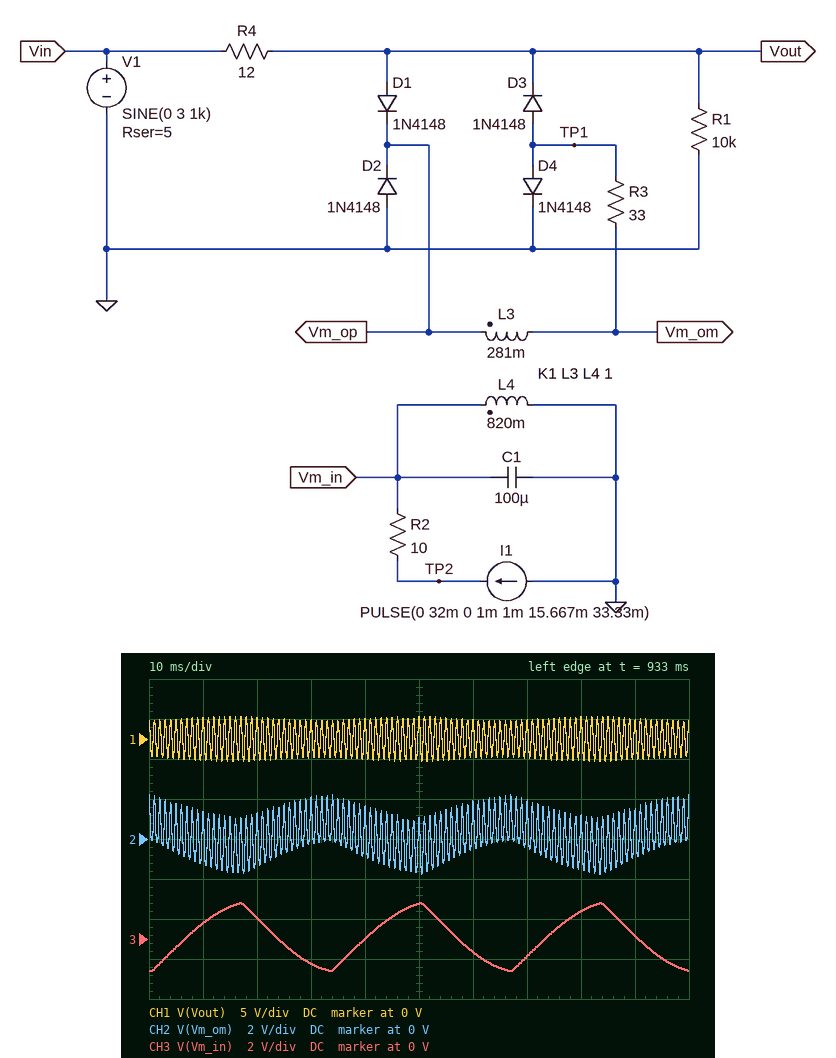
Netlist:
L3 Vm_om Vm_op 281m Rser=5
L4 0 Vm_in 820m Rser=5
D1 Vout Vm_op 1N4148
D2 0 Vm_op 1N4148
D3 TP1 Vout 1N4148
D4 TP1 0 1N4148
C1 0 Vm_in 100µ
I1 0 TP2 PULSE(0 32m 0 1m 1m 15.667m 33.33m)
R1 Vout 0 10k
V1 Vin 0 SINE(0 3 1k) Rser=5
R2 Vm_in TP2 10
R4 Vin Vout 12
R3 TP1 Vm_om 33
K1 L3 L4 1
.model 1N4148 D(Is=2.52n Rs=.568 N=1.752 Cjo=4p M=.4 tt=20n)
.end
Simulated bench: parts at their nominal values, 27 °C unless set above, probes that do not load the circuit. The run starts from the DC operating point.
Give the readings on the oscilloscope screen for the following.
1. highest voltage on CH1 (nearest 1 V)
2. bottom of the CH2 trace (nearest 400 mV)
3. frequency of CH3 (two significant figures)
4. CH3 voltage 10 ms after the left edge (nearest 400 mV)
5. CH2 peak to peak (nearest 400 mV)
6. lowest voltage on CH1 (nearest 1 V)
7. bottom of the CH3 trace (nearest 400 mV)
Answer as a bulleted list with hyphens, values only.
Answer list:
- 3 V
- -1.6 V
- 30 Hz
- 800 mV
- 4.0 V
- -3 V
- -1.6 V
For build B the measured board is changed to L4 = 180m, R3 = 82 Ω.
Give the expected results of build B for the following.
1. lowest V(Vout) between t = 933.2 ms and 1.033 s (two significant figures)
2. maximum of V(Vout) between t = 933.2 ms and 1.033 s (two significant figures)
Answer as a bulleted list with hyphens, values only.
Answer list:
- -3.0 V
- 3.0 V
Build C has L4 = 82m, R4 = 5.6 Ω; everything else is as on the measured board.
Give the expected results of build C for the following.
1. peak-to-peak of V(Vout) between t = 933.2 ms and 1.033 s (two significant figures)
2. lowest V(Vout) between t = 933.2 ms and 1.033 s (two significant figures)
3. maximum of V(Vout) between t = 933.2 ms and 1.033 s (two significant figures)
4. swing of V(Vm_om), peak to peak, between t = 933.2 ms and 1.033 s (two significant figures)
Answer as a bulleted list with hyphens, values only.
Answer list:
- 5.7 V
- -2.9 V
- 2.9 V
- 3.8 V
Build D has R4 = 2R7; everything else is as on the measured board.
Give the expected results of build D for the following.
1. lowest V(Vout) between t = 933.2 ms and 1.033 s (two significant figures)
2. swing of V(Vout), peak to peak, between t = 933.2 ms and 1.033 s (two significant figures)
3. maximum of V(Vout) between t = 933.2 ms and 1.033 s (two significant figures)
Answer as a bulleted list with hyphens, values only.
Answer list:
- -2.9 V
- 5.8 V
- 2.9 V
